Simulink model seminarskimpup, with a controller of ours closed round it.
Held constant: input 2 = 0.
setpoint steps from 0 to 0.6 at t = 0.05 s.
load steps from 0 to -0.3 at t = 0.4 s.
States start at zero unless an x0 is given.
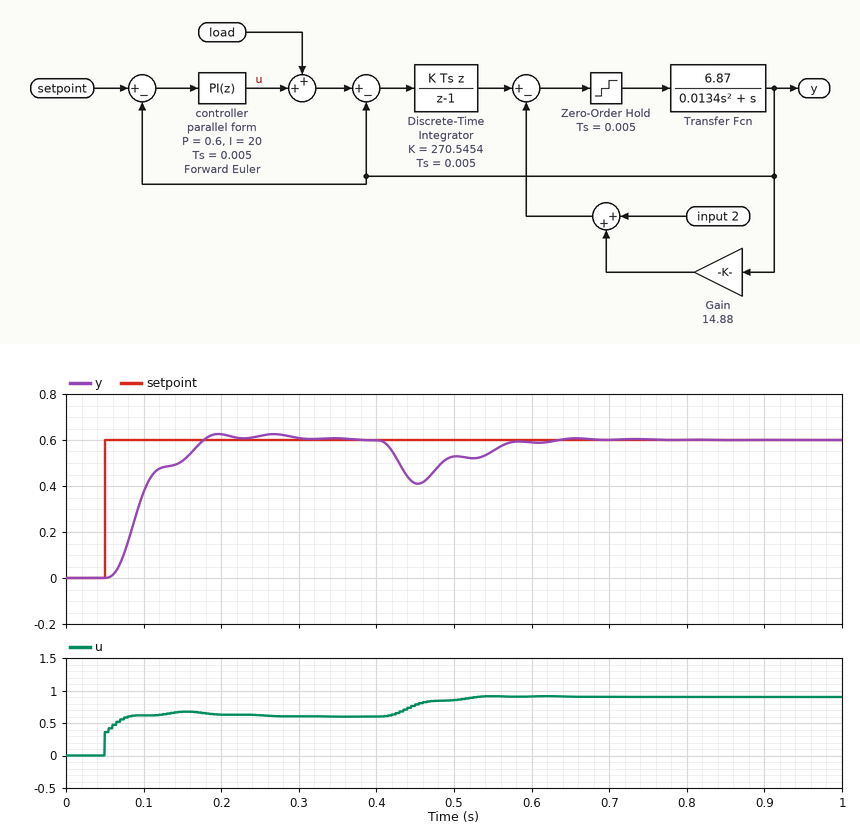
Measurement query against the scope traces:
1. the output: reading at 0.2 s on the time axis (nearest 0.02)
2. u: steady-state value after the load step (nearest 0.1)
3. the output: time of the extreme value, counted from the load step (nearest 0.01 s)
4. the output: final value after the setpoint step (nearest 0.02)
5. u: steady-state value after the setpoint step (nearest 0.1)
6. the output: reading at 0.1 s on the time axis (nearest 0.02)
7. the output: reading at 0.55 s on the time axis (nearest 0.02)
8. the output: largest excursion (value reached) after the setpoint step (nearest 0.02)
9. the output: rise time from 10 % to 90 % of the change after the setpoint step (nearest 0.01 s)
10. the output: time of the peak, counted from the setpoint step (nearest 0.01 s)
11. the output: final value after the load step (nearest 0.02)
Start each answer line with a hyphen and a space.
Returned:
- 0.62
- 0.9
- 0.05 s
- 0.60
- 0.6
- 0.38
- 0.56
- 0.62
- 0.09 s
- 0.15 s
- 0.60
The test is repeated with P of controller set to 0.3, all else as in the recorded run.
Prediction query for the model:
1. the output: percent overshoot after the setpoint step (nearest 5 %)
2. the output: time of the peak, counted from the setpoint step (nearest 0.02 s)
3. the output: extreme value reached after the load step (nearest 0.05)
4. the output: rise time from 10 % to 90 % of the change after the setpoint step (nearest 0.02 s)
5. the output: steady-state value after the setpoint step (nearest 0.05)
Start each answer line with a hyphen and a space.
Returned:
- 10 %
- 0.16 s
- 0.40
- 0.08 s
- 0.60
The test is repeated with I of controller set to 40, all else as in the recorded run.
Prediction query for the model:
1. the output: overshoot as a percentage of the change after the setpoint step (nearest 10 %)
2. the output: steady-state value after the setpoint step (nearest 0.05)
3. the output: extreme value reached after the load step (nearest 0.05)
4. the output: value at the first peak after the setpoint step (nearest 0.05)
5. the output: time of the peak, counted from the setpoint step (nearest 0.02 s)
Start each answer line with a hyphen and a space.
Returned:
- 20 %
- 0.60
- 0.40
- 0.75
- 0.08 s
